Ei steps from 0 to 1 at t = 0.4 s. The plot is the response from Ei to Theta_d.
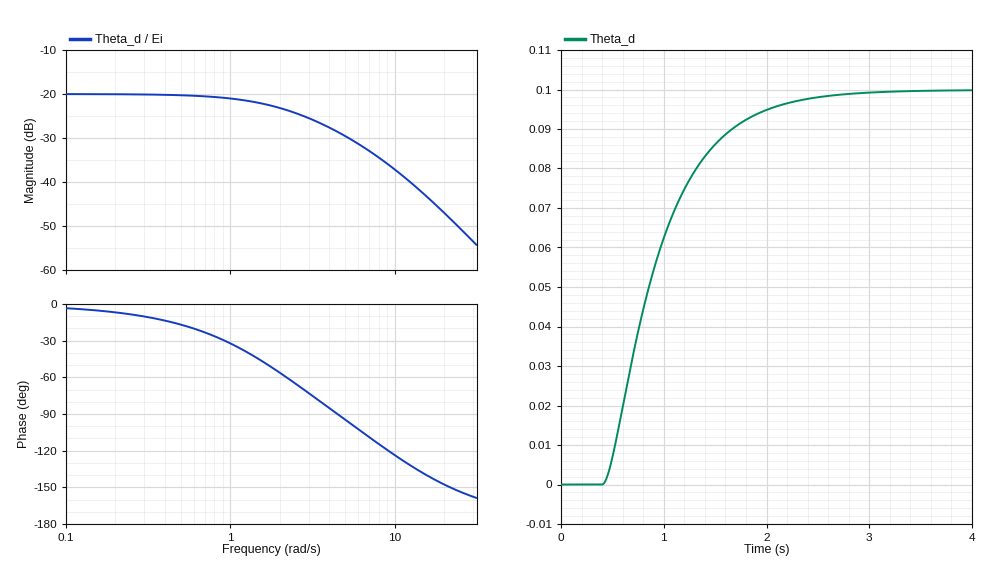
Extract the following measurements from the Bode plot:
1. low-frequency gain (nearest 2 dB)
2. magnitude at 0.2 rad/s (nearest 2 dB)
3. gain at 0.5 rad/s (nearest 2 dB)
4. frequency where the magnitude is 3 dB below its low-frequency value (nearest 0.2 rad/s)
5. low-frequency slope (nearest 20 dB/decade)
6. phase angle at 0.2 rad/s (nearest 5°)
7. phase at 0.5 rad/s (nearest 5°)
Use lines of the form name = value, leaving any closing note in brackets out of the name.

low-frequency gain = -20 dB
magnitude at 0.2 rad/s = -20 dB
gain at 0.5 rad/s = -20 dB
frequency where the magnitude is 3 dB below its low-frequency value = 2.0 rad/s
low-frequency slope = 0 dB/decade
phase angle at 0.2 rad/s = -5°
phase at 0.5 rad/s = -15°
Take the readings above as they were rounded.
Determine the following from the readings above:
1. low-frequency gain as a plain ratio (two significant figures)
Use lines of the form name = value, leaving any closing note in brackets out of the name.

low-frequency gain as a plain ratio = 0.10
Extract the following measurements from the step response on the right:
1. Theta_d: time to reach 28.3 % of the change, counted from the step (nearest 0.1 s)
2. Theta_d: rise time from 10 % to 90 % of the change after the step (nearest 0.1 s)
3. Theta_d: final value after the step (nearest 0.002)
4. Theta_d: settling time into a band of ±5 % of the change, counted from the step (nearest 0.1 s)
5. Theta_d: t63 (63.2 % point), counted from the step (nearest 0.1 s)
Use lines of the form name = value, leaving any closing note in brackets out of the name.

Theta_d: time to reach 28.3 % of the change, counted from the step = 0.3 s
Theta_d: rise time from 10 % to 90 % of the change after the step = 1.1 s
Theta_d: final value after the step = 0.100
Theta_d: settling time into a band of ±5 % of the change, counted from the step = 1.6 s
Theta_d: t63 (63.2 % point), counted from the step = 0.6 s
